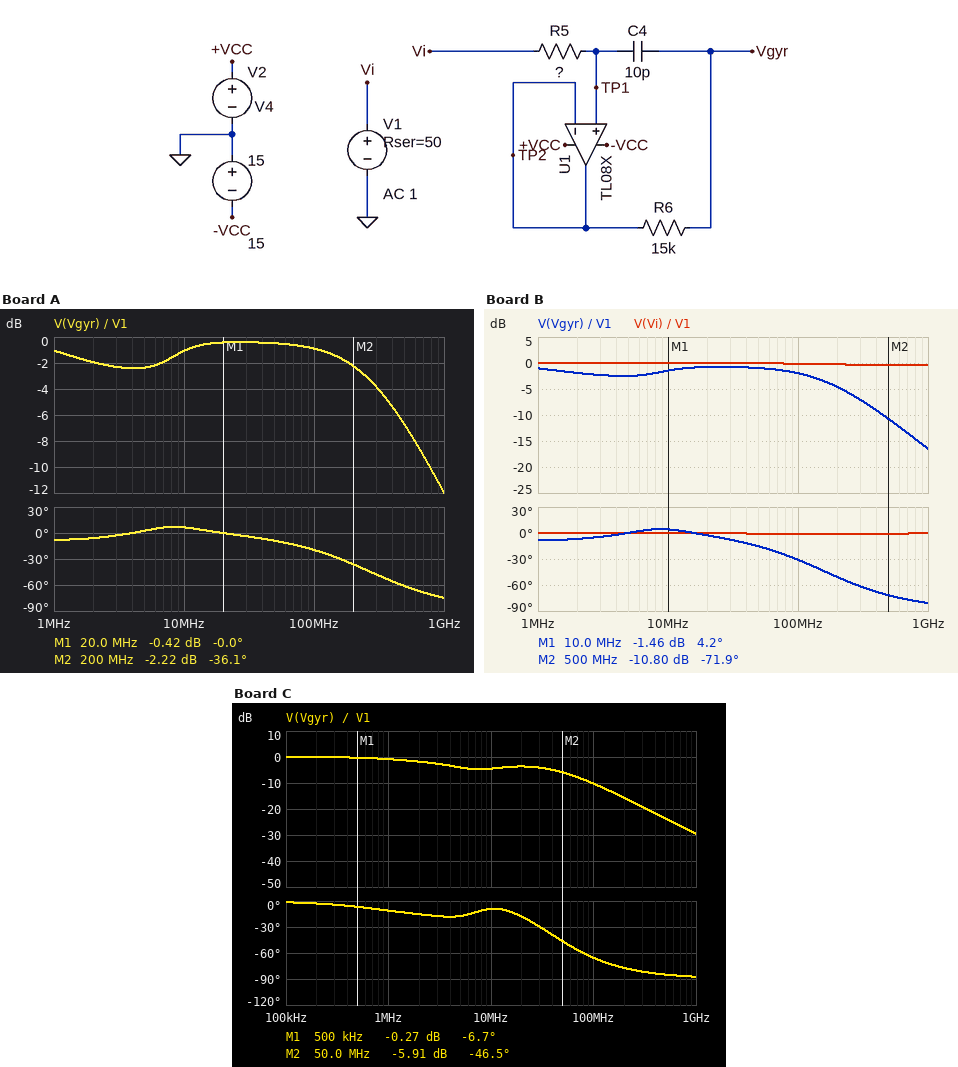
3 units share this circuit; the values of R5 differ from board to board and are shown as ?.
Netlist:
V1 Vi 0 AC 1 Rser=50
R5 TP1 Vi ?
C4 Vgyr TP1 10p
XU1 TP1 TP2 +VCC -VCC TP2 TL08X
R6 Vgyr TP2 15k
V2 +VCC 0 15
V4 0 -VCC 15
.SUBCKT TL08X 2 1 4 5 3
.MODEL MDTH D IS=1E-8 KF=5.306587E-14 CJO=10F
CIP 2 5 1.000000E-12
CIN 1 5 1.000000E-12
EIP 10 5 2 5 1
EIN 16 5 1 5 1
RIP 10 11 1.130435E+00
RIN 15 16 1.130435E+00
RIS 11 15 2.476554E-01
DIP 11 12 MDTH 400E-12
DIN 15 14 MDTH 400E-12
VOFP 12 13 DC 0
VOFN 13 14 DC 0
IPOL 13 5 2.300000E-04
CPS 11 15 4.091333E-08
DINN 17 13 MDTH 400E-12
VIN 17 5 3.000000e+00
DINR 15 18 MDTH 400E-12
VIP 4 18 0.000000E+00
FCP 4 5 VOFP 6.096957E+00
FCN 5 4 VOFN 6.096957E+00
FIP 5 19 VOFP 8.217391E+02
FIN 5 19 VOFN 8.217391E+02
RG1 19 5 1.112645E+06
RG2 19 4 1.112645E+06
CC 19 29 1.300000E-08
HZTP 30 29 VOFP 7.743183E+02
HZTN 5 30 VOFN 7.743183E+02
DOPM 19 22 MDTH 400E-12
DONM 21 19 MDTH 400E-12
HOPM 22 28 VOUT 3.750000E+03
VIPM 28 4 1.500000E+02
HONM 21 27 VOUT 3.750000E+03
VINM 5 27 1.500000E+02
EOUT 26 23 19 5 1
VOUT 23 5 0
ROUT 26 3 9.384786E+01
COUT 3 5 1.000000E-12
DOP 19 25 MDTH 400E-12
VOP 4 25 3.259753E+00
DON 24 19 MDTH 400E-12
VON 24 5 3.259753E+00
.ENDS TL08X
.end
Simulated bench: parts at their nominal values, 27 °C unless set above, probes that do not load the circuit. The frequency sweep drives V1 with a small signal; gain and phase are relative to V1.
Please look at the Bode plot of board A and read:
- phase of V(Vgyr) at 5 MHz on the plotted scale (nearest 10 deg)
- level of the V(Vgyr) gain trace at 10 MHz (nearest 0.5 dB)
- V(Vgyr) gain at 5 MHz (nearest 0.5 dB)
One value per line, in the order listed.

0 deg
-1.0 dB
-2.5 dB
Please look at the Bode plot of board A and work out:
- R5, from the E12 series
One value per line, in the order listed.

560 Ω
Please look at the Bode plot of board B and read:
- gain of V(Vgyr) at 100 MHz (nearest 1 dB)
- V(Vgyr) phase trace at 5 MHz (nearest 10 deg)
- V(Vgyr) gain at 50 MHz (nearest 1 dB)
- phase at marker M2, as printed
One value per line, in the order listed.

-2 dB
0 deg
-1 dB
-71.9 deg
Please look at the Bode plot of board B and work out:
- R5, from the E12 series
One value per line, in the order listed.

1 kΩ
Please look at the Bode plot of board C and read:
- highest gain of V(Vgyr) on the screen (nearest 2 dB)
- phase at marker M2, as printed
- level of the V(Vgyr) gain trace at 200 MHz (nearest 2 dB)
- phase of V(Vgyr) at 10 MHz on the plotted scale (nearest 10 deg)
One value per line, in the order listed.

0 dB
-46.5 deg
-16 dB
-10 deg
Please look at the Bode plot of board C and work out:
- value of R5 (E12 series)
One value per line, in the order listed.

4.7 kΩ
